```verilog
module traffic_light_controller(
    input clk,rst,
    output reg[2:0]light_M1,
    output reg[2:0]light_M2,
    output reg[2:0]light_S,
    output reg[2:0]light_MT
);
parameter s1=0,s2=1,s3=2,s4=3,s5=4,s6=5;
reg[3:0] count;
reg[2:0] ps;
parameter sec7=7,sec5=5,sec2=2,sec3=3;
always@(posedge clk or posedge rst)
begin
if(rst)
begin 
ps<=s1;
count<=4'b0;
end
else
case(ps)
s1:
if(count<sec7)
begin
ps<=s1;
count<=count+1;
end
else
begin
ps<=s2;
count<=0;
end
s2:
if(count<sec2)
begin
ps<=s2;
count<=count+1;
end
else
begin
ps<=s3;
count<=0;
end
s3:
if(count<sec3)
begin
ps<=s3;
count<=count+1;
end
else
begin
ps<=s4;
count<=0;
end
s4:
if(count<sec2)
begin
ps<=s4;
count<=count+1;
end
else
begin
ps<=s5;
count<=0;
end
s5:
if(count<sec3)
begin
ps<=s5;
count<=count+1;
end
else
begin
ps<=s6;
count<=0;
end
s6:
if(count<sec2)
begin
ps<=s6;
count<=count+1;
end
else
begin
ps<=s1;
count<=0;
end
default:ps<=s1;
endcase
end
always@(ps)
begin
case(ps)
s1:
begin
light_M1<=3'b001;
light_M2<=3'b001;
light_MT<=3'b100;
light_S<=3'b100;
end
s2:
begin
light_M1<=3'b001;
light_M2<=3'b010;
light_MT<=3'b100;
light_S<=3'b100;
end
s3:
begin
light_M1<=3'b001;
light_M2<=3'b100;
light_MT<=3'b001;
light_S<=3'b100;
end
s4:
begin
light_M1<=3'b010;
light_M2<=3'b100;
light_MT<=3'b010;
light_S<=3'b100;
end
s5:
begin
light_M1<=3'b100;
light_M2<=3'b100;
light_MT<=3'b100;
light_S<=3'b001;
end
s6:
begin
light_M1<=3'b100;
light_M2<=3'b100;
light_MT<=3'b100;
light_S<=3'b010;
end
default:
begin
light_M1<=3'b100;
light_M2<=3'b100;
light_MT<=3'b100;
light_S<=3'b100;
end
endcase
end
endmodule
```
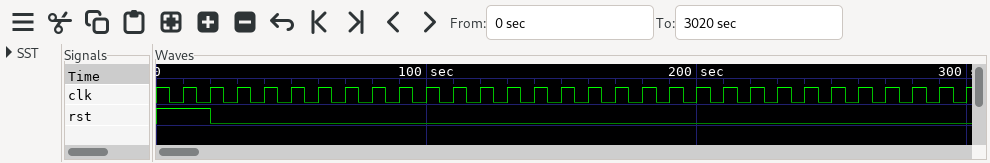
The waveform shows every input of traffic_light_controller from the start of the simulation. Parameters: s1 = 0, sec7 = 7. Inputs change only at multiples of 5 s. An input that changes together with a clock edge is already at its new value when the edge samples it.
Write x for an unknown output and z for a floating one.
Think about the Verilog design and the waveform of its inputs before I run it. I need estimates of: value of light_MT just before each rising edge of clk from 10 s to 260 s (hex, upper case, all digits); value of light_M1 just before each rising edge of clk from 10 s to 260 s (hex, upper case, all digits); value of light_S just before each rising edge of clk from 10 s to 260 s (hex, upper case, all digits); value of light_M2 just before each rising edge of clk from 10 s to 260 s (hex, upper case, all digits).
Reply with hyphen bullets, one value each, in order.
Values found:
- 4, 4, 4, 4, 4, 4, 4, 4, 4, 4, 4, 4, 1, 1, 1, 1, 2, 2, 2, 4, 4, 4, 4, 4, 4, 4
- 1, 1, 1, 1, 1, 1, 1, 1, 1, 1, 1, 1, 1, 1, 1, 1, 2, 2, 2, 4, 4, 4, 4, 4, 4, 4
- 4, 4, 4, 4, 4, 4, 4, 4, 4, 4, 4, 4, 4, 4, 4, 4, 4, 4, 4, 1, 1, 1, 1, 2, 2, 2
- 1, 1, 1, 1, 1, 1, 1, 1, 1, 2, 2, 2, 4, 4, 4, 4, 4, 4, 4, 4, 4, 4, 4, 4, 4, 4
